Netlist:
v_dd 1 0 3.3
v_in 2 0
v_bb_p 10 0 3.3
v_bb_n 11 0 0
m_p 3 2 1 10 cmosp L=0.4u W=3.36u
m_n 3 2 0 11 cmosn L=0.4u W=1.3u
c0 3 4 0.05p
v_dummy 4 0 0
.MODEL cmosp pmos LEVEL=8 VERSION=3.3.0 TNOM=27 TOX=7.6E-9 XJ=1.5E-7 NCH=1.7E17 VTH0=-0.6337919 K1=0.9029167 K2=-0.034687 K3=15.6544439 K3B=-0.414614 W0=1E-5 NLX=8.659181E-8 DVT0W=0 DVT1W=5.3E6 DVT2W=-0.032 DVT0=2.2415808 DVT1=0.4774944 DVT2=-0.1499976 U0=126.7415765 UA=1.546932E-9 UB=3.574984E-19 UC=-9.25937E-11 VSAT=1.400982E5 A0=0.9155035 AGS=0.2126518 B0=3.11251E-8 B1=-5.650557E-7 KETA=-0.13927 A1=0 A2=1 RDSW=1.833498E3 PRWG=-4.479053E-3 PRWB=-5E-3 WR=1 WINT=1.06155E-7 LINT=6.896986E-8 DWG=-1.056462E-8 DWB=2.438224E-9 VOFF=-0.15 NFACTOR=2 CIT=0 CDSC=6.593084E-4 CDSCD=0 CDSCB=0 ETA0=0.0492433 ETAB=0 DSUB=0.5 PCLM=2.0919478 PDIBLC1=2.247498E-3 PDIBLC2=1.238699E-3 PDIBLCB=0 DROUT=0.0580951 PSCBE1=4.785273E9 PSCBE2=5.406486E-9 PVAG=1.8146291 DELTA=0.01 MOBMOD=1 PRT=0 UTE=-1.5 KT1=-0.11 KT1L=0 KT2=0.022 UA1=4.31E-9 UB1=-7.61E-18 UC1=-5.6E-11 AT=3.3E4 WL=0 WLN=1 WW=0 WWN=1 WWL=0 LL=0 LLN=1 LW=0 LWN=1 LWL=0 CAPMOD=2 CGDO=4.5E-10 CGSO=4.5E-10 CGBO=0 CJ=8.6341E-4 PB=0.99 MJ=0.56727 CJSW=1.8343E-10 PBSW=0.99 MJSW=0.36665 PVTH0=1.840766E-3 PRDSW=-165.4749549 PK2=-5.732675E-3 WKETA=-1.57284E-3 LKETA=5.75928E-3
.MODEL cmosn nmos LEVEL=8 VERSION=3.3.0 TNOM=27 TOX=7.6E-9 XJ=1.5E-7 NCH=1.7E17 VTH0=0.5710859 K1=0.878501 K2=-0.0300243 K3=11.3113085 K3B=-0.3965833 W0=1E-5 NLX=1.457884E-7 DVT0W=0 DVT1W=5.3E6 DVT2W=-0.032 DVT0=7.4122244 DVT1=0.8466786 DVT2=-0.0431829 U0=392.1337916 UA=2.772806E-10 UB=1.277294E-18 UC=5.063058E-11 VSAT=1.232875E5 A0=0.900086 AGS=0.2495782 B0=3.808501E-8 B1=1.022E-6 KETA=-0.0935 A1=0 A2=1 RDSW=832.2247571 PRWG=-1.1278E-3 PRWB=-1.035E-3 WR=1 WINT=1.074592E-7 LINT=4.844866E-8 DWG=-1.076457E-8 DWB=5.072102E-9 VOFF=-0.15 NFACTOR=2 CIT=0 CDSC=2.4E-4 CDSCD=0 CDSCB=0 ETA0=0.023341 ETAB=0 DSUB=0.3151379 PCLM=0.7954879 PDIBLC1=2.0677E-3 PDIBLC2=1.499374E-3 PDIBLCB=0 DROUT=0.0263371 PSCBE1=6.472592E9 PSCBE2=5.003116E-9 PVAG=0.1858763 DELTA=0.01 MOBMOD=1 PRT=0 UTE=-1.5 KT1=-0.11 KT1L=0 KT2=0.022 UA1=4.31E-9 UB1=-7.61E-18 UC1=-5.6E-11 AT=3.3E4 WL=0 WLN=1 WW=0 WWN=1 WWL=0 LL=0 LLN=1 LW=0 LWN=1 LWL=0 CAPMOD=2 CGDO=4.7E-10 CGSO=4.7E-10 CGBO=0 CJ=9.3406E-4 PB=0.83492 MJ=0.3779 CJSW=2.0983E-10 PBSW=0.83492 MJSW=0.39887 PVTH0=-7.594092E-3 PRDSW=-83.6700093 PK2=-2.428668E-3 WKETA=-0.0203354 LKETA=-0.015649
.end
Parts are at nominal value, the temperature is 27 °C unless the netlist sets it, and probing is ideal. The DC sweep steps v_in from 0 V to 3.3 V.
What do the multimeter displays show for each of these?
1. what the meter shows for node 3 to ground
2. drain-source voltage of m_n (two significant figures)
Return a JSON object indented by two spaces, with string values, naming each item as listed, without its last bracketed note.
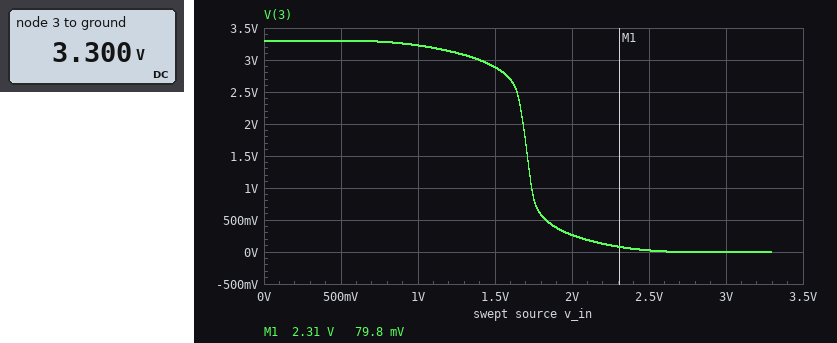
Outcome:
{
  "what the meter shows for node 3 to ground": "3.300 V",
  "drain-source voltage of m_n": "3.3 V"
}
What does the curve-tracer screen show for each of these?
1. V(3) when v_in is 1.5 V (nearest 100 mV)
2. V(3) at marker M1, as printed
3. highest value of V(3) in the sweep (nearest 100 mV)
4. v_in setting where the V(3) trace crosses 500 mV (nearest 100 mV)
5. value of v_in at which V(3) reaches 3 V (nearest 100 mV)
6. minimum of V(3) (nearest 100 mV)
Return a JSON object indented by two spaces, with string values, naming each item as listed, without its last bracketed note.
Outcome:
{
  "V(3) when v_in is 1.5 V": "2.9 V",
  "V(3) at marker M1, as printed": "79.8 mV",
  "highest value of V(3) in the sweep": "3.3 V",
  "v_in setting where the V(3) trace crosses 500 mV": "1.8 V",
  "value of v_in at which V(3) reaches 3 V": "1.4 V",
  "minimum of V(3)": "0 V"
}
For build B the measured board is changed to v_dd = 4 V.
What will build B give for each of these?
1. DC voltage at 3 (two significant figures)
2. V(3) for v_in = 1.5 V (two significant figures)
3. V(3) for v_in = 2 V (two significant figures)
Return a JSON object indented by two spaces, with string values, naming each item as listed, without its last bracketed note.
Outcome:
{
  "DC voltage at 3": "3.9 V",
  "V(3) for v_in = 1.5 V": "3.7 V",
  "V(3) for v_in = 2 V": "3.2 V"
}
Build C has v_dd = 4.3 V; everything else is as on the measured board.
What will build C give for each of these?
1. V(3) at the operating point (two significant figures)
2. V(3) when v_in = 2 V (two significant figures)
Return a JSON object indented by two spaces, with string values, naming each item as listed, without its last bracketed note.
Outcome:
{
  "V(3) at the operating point": "3.9 V",
  "V(3) when v_in = 2 V": "3.7 V"
}
